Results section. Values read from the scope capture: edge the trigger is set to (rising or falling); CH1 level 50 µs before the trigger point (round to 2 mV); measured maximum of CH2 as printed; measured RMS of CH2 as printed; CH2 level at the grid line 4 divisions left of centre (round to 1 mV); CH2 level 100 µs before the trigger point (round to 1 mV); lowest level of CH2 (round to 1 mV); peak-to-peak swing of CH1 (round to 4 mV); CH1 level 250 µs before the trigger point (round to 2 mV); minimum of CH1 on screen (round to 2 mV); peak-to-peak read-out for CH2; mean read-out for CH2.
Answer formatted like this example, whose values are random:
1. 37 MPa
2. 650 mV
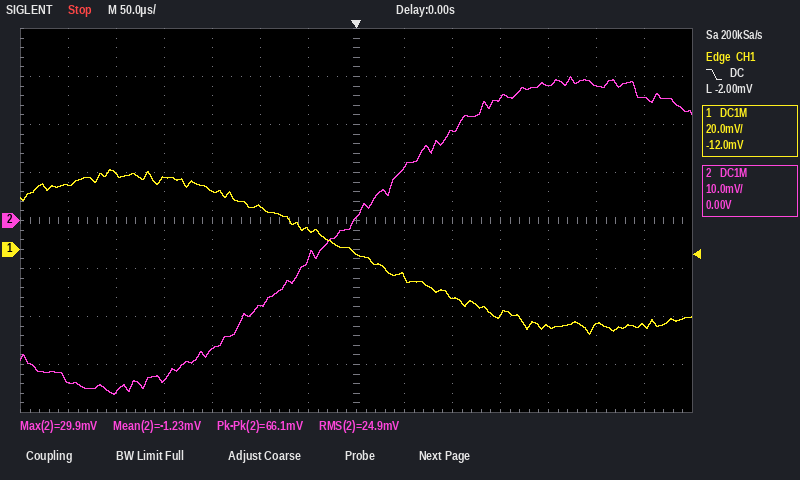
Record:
1. falling
2. 8 mV
3. 29.9 mV
4. 24.9 mV
5. -33 mV
6. -18 mV
7. -36 mV
8. 68 mV
9. 32 mV
10. -36 mV
11. 66.1 mV
12. -1.23 mV
